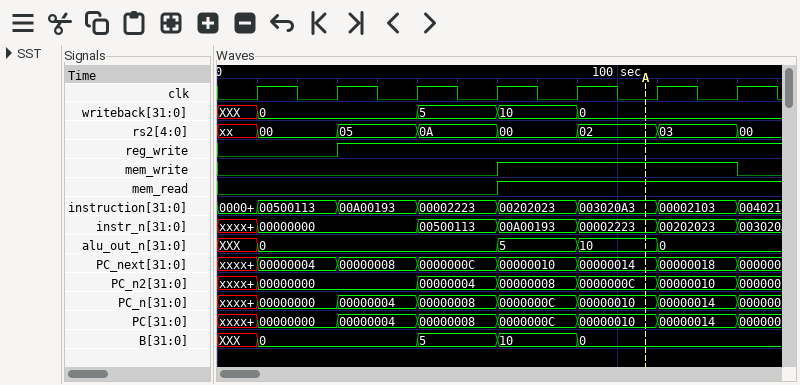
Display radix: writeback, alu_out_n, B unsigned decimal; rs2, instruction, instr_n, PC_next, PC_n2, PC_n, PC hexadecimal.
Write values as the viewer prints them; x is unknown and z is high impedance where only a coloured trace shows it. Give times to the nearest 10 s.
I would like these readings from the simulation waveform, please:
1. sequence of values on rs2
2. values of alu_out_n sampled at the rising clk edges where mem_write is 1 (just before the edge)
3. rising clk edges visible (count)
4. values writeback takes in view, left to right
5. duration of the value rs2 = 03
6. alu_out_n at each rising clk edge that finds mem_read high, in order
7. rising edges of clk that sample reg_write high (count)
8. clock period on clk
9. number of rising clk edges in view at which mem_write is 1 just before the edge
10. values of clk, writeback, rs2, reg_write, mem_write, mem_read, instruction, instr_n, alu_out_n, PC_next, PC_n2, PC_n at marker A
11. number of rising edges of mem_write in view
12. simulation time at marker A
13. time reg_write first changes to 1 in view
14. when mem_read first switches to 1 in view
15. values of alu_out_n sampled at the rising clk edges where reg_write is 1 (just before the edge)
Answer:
xx, 00, 05, 0A, 00, 02, 03, 00
5, 10, 0
7
XXX, 0, 5, 10, 0
20 s
5, 10, 0
5
20 s
3
clk=0, writeback=0, rs2=02, reg_write=1, mem_write=1, mem_read=1, instruction=003020A3, instr_n=00002223, alu_out_n=10, PC_next=00000014, PC_n2=0000000C, PC_n=00000010
1
110 s
30 s
70 s
0, 0, 5, 10, 0
